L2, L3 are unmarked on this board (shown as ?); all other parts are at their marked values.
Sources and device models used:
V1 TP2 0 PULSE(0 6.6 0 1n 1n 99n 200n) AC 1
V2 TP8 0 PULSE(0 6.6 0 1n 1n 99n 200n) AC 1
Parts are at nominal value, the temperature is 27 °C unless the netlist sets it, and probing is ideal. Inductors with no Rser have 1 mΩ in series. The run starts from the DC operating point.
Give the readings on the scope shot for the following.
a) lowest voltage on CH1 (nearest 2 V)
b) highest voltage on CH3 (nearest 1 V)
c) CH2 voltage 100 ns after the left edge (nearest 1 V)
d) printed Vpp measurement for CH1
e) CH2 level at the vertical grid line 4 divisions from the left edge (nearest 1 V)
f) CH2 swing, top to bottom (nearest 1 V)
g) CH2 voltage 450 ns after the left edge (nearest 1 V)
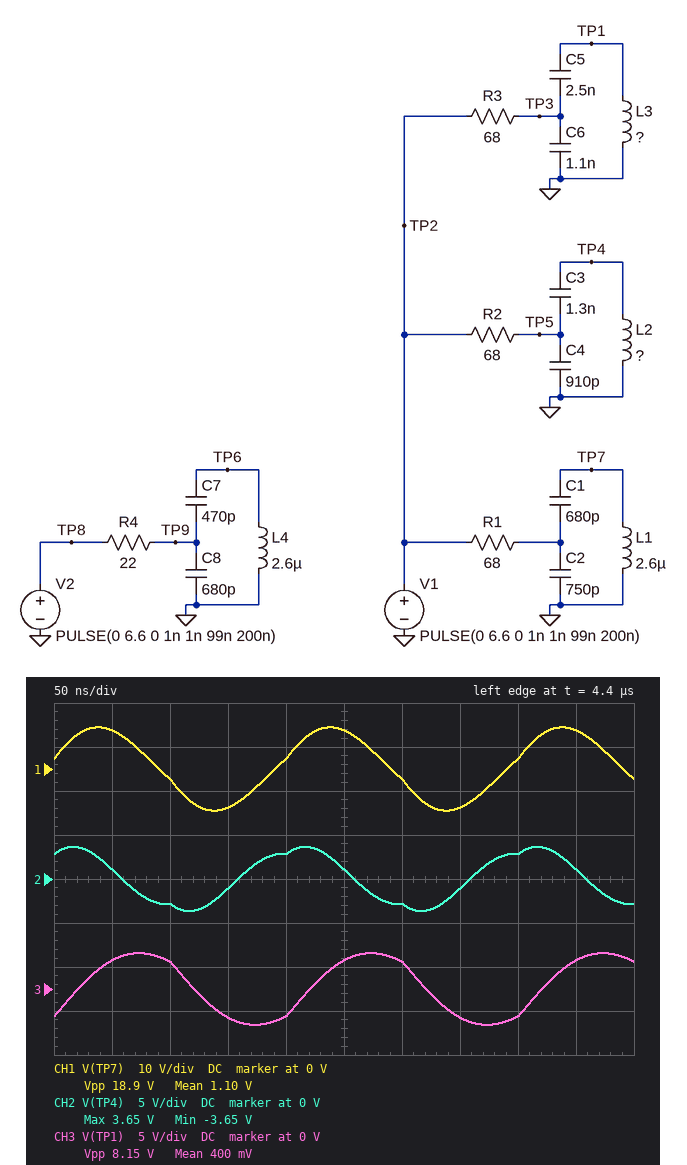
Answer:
-10 V
4 V
-3 V
18.9 V
3 V
7 V
1 V
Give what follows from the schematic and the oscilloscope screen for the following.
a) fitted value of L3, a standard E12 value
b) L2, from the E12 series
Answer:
1.8 µH
1.2 µH
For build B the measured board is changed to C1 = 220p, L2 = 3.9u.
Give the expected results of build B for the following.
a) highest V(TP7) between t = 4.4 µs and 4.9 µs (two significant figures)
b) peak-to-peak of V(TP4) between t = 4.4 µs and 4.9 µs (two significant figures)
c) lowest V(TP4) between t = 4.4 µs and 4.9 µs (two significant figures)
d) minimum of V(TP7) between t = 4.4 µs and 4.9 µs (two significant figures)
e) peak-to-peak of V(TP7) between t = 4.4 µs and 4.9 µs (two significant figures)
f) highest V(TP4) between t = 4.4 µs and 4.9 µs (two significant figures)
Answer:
2.0 V
6.4 V
-3.2 V
-2.0 V
4.0 V
3.2 V
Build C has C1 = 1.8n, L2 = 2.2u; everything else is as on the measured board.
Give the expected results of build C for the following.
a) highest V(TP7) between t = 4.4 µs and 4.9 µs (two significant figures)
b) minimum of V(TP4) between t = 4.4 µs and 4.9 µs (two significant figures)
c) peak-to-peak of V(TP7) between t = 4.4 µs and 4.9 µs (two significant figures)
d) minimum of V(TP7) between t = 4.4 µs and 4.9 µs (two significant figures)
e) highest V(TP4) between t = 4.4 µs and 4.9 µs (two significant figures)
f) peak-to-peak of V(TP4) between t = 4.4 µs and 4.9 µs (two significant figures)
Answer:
4.5 V
-5.8 V
8.9 V
-4.5 V
5.8 V
12 V
